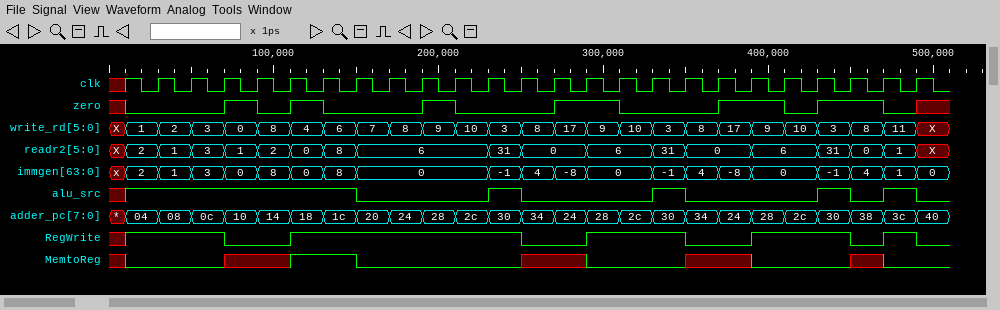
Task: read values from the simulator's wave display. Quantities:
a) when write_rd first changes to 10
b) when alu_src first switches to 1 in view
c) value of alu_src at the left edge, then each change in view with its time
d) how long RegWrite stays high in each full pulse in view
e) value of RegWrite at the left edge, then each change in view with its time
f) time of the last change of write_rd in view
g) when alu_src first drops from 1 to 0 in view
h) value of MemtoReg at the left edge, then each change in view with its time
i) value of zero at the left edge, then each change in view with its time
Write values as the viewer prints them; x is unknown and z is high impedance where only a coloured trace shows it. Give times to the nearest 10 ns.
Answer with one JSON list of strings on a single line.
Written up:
["210 ns", "10 ns", "x, 1 at 10 ns, 0 at 150 ns, 1 at 230 ns, 0 at 250 ns, 1 at 330 ns, 0 at 350 ns, 1 at 430 ns, 0 at 450 ns, 1 at 470 ns, 0 at 490 ns", "140 ns, 60 ns, 60 ns, 20 ns", "x, 1 at 10 ns, 0 at 70 ns, 1 at 110 ns, 0 at 250 ns, 1 at 290 ns, 0 at 350 ns, 1 at 390 ns, 0 at 450 ns, 1 at 470 ns, 0 at 490 ns", "490 ns", "150 ns", "x, 0 at 10 ns, x at 70 ns, 1 at 110 ns, 0 at 150 ns, x at 250 ns, 0 at 290 ns, x at 350 ns, 0 at 390 ns, x at 450 ns, 0 at 470 ns", "x, 0 at 10 ns, 1 at 70 ns, 0 at 90 ns, 1 at 110 ns, 0 at 130 ns, 1 at 190 ns, 0 at 210 ns, 1 at 270 ns, 0 at 310 ns, 1 at 370 ns, 0 at 410 ns, 1 at 430 ns, 0 at 470 ns, x at 490 ns"]
